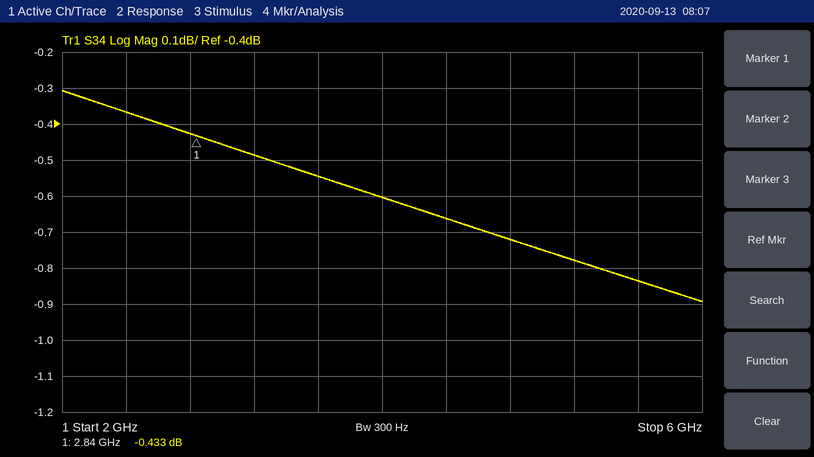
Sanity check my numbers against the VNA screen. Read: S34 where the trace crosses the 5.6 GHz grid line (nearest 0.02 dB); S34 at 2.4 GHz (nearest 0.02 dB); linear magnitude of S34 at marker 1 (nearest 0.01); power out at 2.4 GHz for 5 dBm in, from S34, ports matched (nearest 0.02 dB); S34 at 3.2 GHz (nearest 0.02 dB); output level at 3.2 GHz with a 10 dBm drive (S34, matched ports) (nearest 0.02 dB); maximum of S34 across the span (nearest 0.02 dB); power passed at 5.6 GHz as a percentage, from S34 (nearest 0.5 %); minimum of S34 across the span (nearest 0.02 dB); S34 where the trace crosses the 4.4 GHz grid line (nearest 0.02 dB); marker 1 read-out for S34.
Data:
-0.84 dB
-0.36 dB
0.95
4.64 dBm
-0.48 dB
9.52 dBm
-0.30 dB
82.5 %
-0.90 dB
-0.66 dB
-0.433 dB
